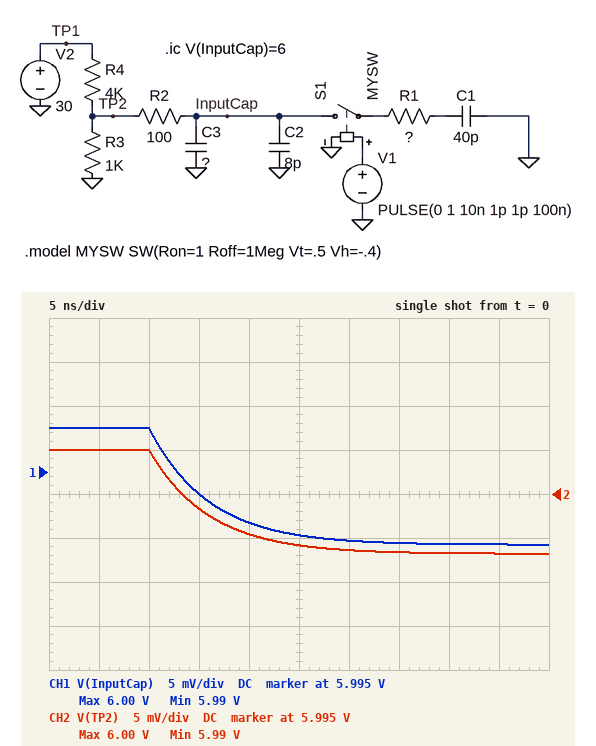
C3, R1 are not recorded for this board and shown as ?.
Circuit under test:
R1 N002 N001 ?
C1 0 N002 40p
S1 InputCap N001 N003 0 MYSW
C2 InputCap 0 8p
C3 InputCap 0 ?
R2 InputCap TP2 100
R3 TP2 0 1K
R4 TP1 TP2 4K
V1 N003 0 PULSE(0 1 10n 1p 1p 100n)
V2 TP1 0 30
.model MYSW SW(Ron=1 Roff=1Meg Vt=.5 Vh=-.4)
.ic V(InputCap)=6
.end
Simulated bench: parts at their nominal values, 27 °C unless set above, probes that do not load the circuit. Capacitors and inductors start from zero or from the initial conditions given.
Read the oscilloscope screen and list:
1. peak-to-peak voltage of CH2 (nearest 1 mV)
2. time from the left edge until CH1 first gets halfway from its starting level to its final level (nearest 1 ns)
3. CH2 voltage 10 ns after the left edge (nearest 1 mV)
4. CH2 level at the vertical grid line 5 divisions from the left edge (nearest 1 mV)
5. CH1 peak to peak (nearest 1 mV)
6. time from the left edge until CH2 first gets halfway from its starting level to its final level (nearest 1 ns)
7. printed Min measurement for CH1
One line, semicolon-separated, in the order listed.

12 mV; 14 ns; 6.000 V; 5.989 V; 13 mV; 14 ns; 5.99 V
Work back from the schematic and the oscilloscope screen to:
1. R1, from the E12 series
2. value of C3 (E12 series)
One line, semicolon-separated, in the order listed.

150 Ω; 18 nF
